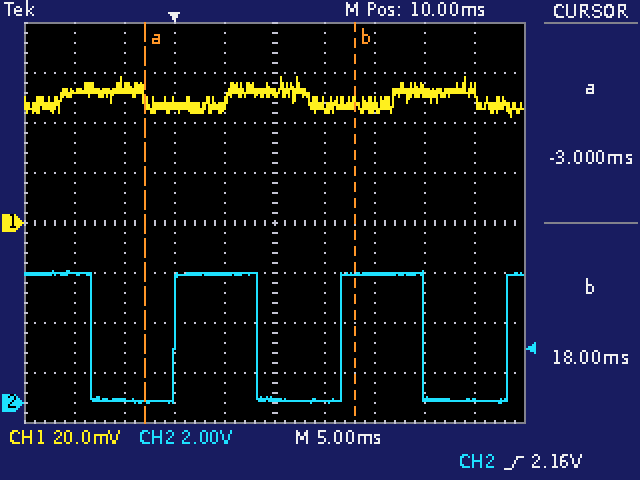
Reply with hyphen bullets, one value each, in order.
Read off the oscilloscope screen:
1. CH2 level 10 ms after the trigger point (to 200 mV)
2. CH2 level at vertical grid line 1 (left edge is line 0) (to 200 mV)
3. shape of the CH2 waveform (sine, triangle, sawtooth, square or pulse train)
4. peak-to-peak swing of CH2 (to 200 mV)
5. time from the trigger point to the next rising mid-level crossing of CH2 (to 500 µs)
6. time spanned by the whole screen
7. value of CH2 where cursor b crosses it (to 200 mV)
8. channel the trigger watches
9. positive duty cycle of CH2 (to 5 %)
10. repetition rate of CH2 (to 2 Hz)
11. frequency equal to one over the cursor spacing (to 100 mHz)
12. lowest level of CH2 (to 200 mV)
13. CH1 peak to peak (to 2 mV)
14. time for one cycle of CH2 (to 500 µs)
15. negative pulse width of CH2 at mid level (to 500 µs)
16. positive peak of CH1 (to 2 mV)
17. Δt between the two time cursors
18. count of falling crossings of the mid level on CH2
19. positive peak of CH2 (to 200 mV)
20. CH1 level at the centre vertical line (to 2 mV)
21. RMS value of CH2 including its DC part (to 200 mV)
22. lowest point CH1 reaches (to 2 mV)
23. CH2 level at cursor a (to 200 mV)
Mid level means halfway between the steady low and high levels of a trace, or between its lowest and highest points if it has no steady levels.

- 200 mV
- 5.2 V
- square
- 5.2 V
- 16.5 ms
- 50 ms
- 5.2 V
- CH2
- 50 %
- 60 Hz
- 47.6 Hz
- 0.0 V
- 16 mV
- 16.5 ms
- 8.5 ms
- 58 mV
- 21.0 ms
- 3
- 5.2 V
- 52 mV
- 3.6 V
- 42 mV
- 0.0 V
